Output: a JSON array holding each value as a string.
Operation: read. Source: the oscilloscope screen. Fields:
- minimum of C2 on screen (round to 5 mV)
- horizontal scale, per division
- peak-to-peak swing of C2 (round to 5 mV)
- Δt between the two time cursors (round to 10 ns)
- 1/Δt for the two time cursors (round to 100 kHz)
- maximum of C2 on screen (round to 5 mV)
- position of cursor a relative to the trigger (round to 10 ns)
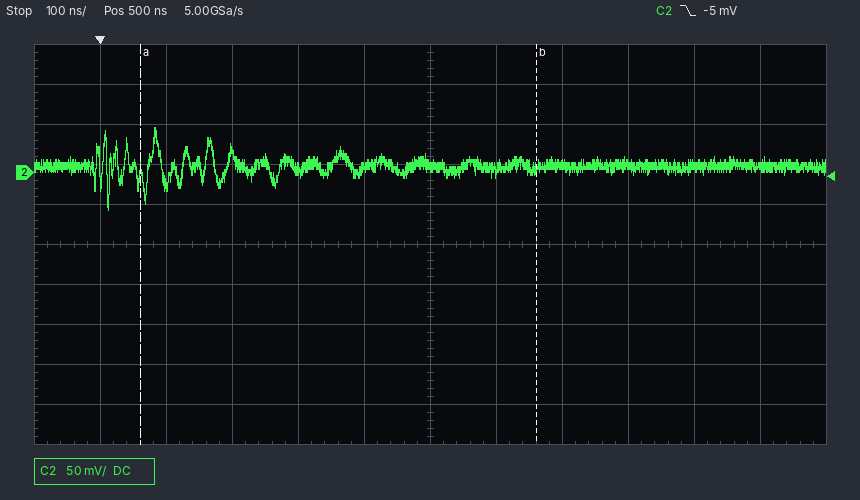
["-50 mV", "100 ns", "105 mV", "600 ns", "1.7 MHz", "55 mV", "+60 ns"]
